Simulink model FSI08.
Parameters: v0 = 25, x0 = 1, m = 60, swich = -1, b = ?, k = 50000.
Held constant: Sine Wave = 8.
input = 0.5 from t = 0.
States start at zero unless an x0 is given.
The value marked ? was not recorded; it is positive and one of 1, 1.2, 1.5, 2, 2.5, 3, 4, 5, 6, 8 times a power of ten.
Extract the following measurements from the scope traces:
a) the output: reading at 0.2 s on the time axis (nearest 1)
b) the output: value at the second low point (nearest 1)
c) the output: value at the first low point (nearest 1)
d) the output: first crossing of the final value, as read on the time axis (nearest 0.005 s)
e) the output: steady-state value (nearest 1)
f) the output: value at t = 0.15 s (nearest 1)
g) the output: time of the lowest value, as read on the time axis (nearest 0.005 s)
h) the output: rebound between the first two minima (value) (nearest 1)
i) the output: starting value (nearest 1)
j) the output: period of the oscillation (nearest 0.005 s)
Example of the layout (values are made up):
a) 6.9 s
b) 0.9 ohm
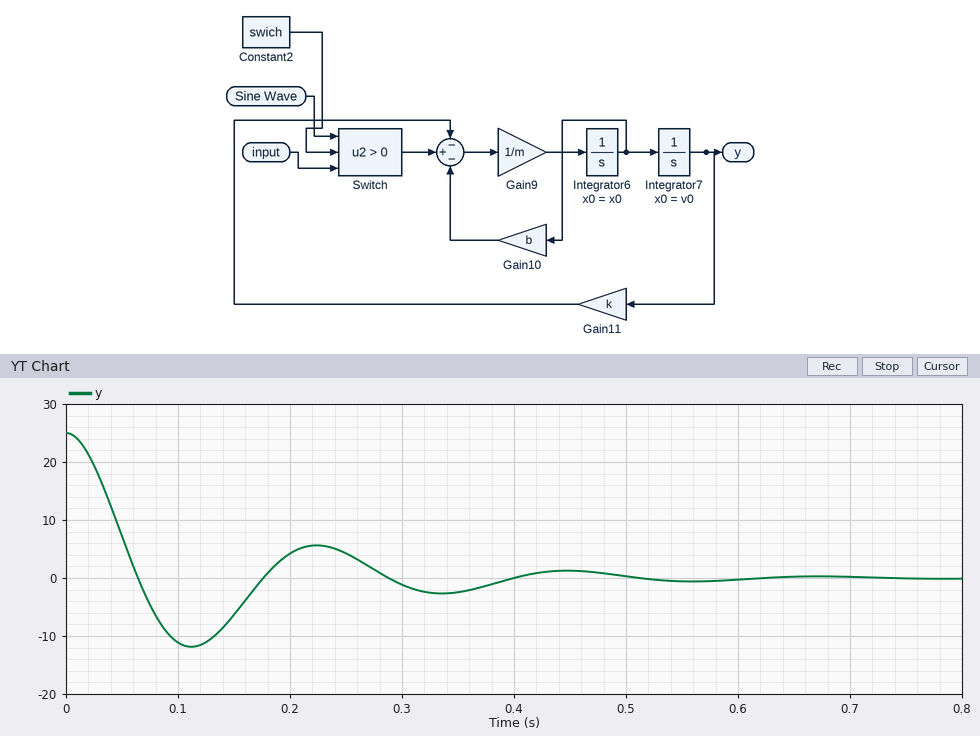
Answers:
a) 4
b) -3
c) -12
d) 0.065 s
e) 0
f) -6
g) 0.110 s
h) 6
i) 25
j) 0.225 s
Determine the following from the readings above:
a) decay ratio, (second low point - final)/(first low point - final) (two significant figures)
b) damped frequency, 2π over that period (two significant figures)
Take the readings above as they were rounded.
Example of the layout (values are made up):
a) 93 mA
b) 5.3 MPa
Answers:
a) 0.25
b) 28 rad/s
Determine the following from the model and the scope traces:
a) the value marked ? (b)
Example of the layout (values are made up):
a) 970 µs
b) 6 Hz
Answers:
a) 800
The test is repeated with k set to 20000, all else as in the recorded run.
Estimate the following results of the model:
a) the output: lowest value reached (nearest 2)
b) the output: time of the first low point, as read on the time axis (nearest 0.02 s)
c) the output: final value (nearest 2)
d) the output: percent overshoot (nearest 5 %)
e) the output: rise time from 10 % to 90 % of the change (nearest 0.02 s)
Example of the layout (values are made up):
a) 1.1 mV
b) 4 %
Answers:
a) -8
b) 0.18 s
c) 0
d) 30 %
e) 0.08 s
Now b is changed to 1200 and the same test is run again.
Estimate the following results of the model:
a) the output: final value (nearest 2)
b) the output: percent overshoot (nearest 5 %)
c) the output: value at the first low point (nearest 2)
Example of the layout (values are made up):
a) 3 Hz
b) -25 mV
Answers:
a) 0
b) 30 %
c) -8
